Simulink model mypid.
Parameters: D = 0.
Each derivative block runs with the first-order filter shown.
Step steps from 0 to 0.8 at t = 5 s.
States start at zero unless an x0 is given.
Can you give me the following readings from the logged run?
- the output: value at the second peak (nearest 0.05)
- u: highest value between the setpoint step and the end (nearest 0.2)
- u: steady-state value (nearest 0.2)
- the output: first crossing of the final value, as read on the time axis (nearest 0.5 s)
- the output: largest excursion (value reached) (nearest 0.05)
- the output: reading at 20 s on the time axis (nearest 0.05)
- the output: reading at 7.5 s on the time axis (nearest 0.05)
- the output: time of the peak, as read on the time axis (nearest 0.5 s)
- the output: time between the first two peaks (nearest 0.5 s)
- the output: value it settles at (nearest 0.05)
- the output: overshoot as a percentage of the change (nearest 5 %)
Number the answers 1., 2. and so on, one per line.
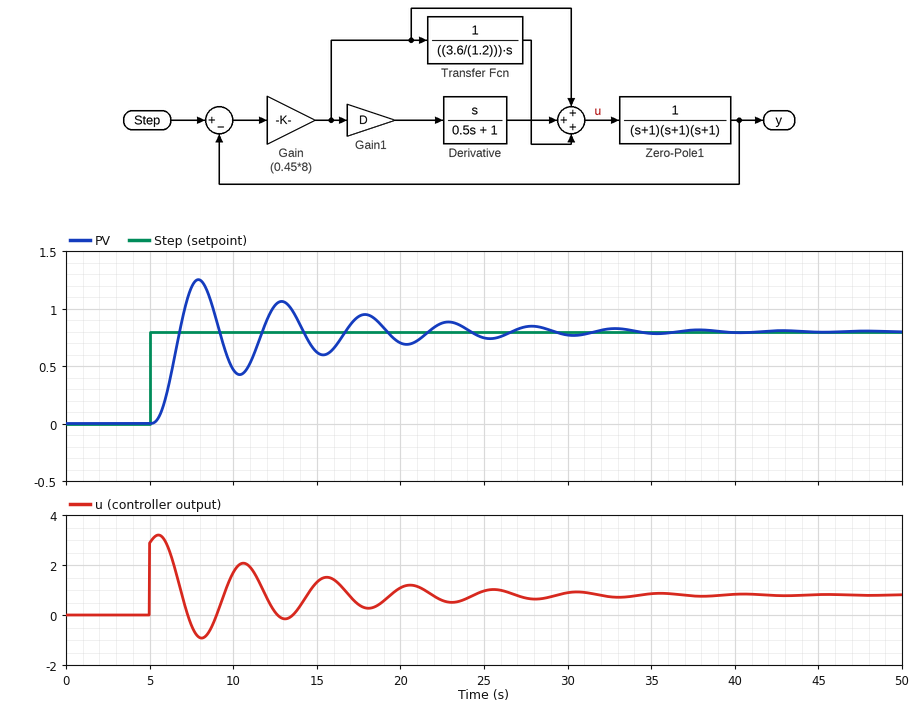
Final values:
1. 1.05
2. 3.2
3. 0.8
4. 7.0 s
5. 1.25
6. 0.70
7. 1.20
8. 8.0 s
9. 5.0 s
10. 0.80
11. 55 %
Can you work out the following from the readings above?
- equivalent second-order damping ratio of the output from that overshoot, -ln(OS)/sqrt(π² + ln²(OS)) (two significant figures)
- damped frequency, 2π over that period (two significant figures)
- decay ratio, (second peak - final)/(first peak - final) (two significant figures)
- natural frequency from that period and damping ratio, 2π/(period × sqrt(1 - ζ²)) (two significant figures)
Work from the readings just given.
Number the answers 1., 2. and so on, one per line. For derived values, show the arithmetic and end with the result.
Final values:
1. ln(0.55) = -0.598; 0.598 / sqrt(9.870 + 0.357) = 0.19
2. 2π / 5 = 1.3 rad/s
3. (1.05 - 0.8) / (1.25 - 0.8) = 0.56
4. 2π / (5 × sqrt(1 - 0.19²)) = 1.3 rad/s
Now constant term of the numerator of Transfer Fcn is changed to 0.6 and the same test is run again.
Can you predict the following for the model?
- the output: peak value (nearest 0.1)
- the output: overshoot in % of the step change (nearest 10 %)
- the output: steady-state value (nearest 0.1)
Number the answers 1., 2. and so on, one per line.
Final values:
1. 1.1
2. 40 %
3. 0.8
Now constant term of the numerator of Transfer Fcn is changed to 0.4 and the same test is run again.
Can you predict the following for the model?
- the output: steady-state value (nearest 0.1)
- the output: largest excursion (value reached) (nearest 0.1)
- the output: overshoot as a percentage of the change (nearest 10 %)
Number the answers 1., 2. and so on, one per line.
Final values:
1. 0.8
2. 1.1
3. 30 %
